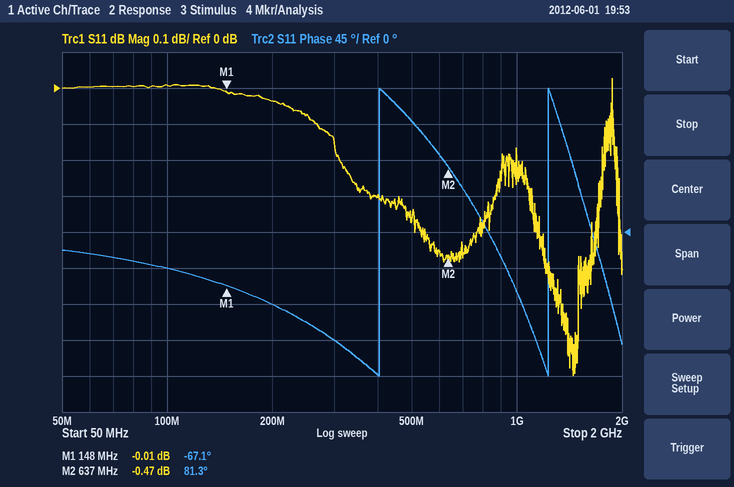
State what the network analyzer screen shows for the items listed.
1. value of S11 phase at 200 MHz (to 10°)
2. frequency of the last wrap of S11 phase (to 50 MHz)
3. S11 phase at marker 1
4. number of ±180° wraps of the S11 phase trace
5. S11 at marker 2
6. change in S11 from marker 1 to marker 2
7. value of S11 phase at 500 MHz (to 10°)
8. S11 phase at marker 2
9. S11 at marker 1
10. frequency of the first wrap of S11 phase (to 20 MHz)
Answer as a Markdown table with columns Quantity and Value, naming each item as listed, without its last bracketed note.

| Quantity | Value |
|---|---|
| value of S11 phase at 200 MHz | -90° |
| frequency of the last wrap of S11 phase | 1.25 GHz |
| S11 phase at marker 1 | -67.1° |
| number of ±180° wraps of the S11 phase trace | 2 |
| S11 at marker 2 | -0.47 dB |
| change in S11 from marker 1 to marker 2 | -0.46 dB |
| value of S11 phase at 500 MHz | 140° |
| S11 phase at marker 2 | 81.3° |
| S11 at marker 1 | -0.01 dB |
| frequency of the first wrap of S11 phase | 400 MHz |
